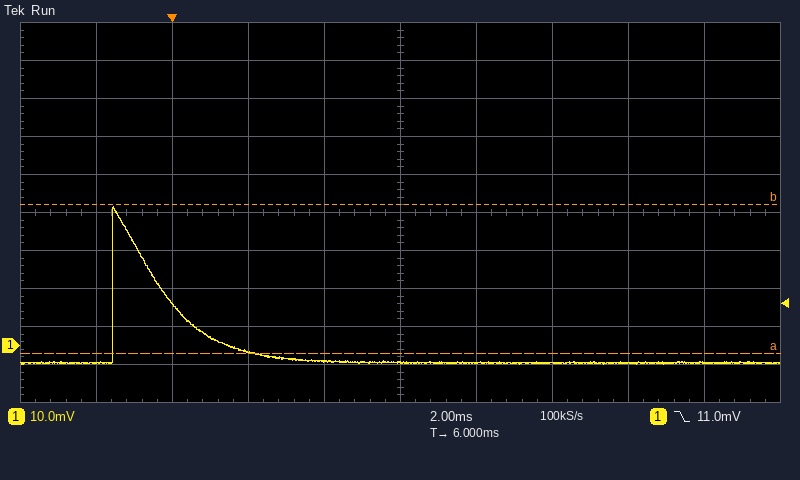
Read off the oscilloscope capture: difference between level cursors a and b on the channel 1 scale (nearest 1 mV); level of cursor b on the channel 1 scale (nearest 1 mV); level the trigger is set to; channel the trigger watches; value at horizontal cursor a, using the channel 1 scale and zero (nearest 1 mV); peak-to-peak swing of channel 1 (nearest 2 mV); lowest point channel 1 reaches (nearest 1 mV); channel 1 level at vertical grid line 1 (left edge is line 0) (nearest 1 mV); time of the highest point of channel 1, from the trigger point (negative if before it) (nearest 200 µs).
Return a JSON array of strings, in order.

["39 mV", "37 mV", "11.0 mV", "channel 1", "-2 mV", "42 mV", "-5 mV", "-5 mV", "-1.6 ms"]
